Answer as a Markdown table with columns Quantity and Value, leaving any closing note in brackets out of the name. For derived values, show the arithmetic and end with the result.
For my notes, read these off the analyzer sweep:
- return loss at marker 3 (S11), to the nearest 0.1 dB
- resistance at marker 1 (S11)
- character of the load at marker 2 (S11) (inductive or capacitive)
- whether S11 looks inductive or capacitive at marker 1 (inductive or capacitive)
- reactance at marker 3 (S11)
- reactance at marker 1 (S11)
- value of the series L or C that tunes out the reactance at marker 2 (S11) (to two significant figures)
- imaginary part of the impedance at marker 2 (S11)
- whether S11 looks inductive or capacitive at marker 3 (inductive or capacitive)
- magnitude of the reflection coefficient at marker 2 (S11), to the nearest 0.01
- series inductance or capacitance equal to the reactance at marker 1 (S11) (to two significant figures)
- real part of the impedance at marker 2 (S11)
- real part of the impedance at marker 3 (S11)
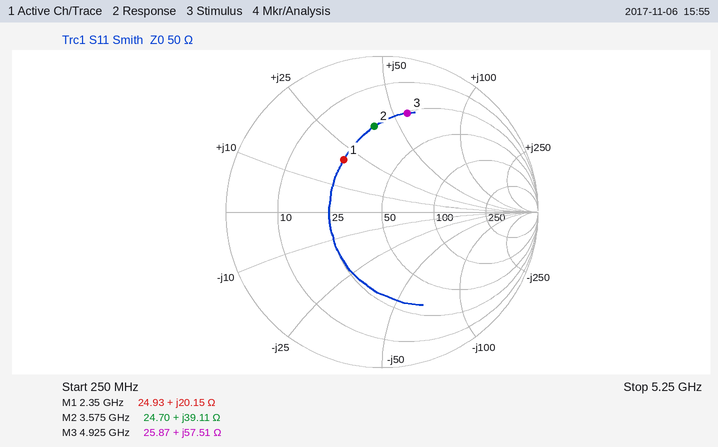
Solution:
| Quantity | Value |
|---|---|
| return loss at marker 3 (S11), to the nearest 0.1 dB | 3.7 dB |
| resistance at marker 1 | 24.93 Ω |
| character of the load at marker 2 (S11) | inductive |
| whether S11 looks inductive or capacitive at marker 1 | inductive |
| reactance at marker 3 | +57.51 Ω |
| reactance at marker 1 | +20.15 Ω |
| value of the series L or C that tunes out the reactance at marker 2 (S11) | C = 1/(2π × 3.575 GHz × 39.11 Ω) ≈ 1.1 pF |
| imaginary part of the impedance at marker 2 | +39.11 Ω |
| whether S11 looks inductive or capacitive at marker 3 | inductive |
| magnitude of the reflection coefficient at marker 2 (S11), to the nearest 0.01 | 0.55 |
| series inductance or capacitance equal to the reactance at marker 1 (S11) | L = 20.15 Ω/(2π × 2.35 GHz) ≈ 1.4 nH |
| real part of the impedance at marker 2 | 24.70 Ω |
| real part of the impedance at marker 3 | 25.87 Ω |
